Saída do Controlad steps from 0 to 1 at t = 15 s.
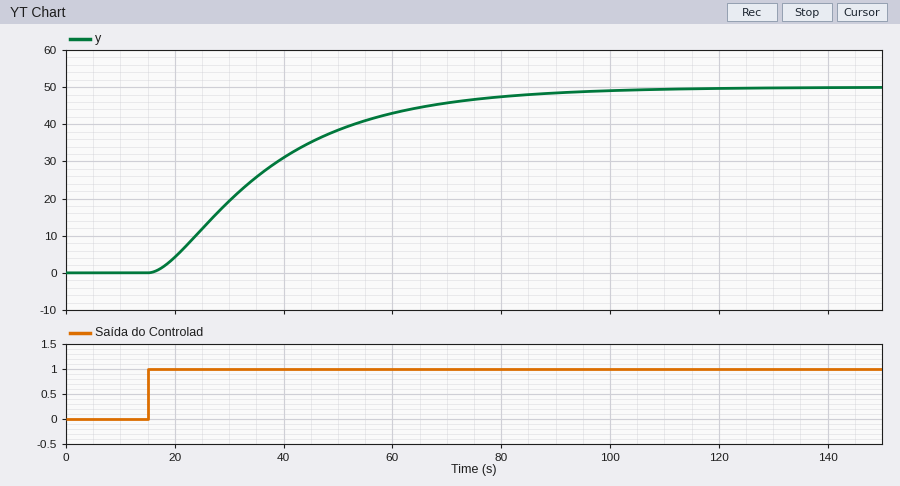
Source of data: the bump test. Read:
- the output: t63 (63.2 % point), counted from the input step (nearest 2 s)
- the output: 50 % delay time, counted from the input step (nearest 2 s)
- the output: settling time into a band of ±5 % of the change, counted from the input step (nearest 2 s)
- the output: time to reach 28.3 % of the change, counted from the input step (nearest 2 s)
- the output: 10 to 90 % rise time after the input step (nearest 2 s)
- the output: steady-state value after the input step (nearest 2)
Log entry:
26 s
20 s
66 s
12 s
46 s
50
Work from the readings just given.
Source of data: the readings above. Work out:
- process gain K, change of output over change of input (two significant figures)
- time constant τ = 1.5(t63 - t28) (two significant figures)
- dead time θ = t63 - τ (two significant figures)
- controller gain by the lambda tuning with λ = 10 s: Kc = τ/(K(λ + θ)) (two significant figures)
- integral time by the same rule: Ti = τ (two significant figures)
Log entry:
50
21 s
5.0 s
0.028
21 s
